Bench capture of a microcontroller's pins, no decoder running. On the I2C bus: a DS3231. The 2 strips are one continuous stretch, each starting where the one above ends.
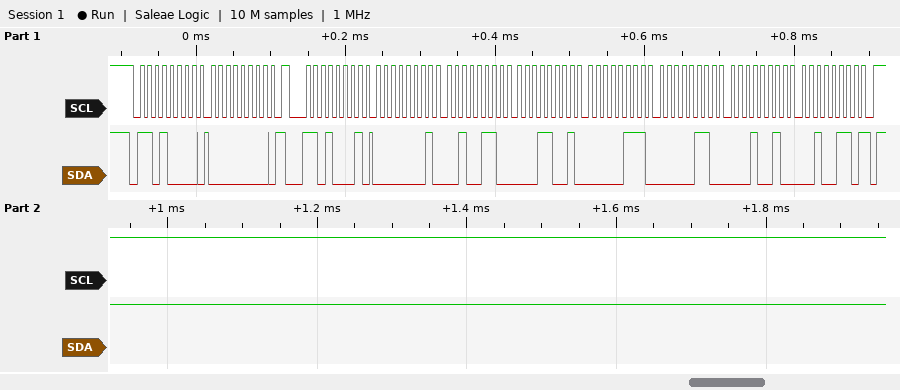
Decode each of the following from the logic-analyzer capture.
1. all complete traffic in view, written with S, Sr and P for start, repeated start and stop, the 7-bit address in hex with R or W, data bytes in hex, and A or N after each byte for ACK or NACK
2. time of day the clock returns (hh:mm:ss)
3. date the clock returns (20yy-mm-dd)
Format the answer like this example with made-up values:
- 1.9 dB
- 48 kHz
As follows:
- S 68W A 00 A Sr 68R A 01 A 26 A 19 A 07 A 06 A 12 A 26 N P
- 19:26:01
- 2026-12-06
